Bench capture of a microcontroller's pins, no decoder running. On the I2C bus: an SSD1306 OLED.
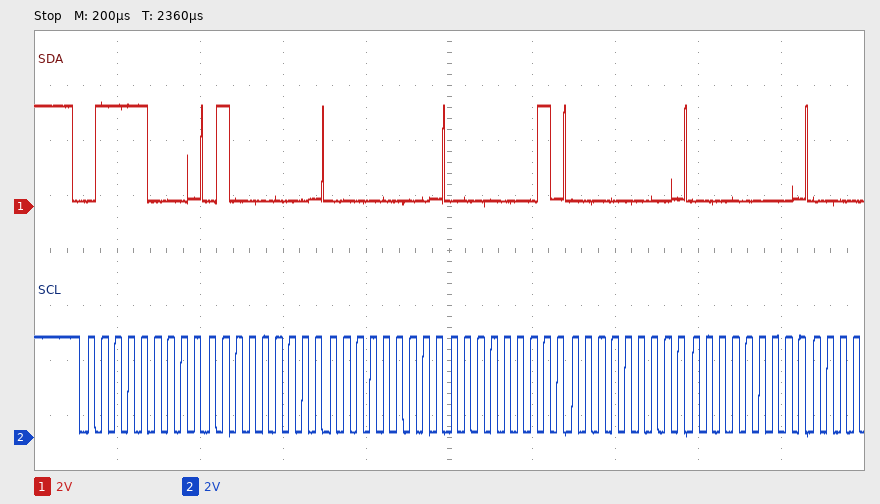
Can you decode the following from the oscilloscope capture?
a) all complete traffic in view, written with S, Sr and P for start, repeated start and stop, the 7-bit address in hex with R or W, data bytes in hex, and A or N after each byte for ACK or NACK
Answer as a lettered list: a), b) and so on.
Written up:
a) S 3CW A 40 A 00 A 01 A 00 A 00 A
